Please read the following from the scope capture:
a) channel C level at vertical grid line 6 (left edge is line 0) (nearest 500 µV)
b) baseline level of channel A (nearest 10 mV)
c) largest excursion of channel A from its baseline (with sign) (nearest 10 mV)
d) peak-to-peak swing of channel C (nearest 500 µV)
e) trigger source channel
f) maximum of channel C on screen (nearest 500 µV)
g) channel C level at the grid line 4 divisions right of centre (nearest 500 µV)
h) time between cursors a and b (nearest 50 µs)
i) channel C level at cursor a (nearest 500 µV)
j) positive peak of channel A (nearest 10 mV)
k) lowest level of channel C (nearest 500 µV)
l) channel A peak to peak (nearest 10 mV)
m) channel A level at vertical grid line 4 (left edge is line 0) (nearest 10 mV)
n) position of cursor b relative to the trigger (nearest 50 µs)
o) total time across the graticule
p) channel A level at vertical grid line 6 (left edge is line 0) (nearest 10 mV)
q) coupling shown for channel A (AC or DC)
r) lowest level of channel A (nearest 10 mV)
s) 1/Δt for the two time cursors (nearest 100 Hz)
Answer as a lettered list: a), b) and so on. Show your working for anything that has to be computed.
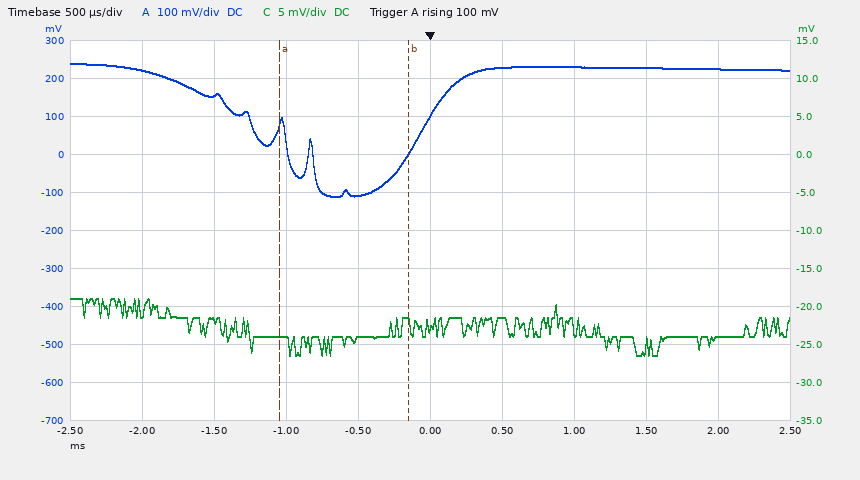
a) -21.5 mV
b) 230 mV
c) -110 mV − (230 mV) = -340 mV
d) -19.0 mV − (-26.5 mV) = 7.5 mV
e) channel A
f) -19.0 mV
g) -24.0 mV
h) 900 µs
i) -24.0 mV
j) 240 mV
k) -26.5 mV
l) 240 mV − (-110 mV) = 350 mV
m) -110 mV
n) -150 µs
o) 5 ms
p) 230 mV
q) DC
r) -110 mV
s) 1 / 900 µs ≈ 1.1 kHz
